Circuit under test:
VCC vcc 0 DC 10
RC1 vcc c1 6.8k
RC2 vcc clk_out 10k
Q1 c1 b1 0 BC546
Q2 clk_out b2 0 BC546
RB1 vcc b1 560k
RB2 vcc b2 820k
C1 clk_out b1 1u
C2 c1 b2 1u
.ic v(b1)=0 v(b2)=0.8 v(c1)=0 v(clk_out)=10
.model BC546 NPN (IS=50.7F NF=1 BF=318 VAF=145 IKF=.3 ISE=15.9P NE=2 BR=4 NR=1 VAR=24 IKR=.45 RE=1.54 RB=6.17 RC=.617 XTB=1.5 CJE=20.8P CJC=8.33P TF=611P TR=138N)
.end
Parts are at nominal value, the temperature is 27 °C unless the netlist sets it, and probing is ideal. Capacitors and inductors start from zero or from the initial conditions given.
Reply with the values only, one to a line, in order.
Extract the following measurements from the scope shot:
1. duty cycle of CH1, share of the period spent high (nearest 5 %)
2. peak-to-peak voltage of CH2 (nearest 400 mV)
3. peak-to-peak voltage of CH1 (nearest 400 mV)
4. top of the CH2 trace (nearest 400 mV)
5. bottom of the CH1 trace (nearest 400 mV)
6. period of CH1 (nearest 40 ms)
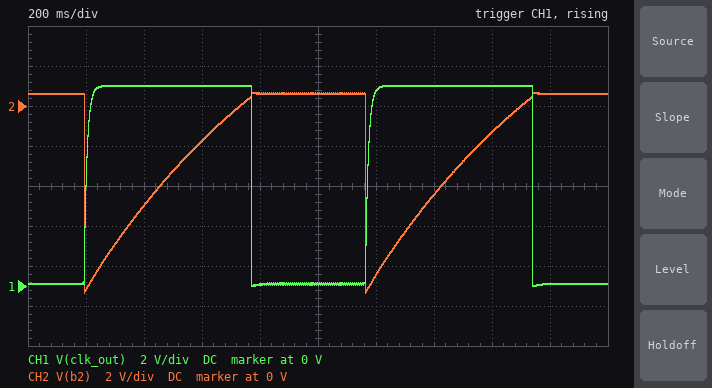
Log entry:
60 %
10.0 V
10.0 V
800 mV
0 V
960 ms
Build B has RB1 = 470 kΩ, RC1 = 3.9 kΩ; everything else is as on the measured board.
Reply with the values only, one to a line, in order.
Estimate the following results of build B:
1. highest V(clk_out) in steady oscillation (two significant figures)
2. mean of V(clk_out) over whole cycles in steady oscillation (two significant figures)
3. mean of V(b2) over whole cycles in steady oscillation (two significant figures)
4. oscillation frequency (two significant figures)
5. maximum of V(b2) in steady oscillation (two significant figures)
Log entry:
10 V
6.3 V
-2.2 V
1.1 Hz
700 mV
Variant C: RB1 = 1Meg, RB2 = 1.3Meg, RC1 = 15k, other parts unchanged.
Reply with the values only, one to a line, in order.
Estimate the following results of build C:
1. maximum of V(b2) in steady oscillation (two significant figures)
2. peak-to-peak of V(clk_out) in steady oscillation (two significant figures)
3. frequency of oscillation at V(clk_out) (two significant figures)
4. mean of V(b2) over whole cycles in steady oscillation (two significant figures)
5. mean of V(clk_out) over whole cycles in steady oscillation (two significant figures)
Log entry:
660 mV
10 V
620 mHz
-1.9 V
5.7 V
